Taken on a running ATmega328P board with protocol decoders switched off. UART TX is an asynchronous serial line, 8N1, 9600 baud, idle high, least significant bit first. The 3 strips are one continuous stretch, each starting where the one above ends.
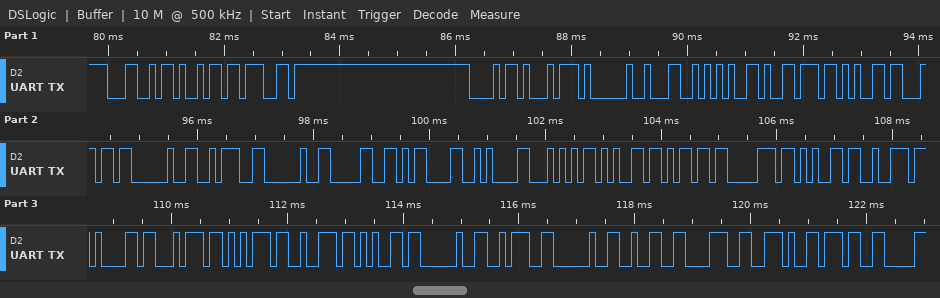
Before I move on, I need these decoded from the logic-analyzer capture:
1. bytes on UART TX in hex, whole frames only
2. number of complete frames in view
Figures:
4C 69 67 68 74 20 4C 65 76 65 6C 20 3A 20 30 0D 0A 54 65 6D 70 65 72 61 74 75 72 65 20 3A 20 32 38 2E 37
35
